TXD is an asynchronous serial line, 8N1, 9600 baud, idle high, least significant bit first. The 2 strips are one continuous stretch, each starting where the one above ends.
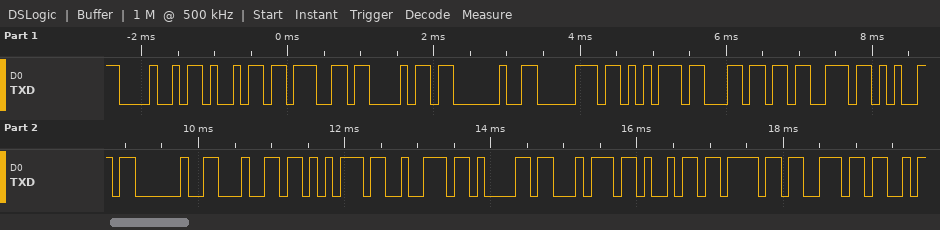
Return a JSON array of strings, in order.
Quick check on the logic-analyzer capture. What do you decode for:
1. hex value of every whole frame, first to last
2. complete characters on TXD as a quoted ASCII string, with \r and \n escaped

["48 69 67 68 20 70 75 6C 73 65 20 64 75 72 61 74 69 6F 6E", "\"High pulse duration\""]
